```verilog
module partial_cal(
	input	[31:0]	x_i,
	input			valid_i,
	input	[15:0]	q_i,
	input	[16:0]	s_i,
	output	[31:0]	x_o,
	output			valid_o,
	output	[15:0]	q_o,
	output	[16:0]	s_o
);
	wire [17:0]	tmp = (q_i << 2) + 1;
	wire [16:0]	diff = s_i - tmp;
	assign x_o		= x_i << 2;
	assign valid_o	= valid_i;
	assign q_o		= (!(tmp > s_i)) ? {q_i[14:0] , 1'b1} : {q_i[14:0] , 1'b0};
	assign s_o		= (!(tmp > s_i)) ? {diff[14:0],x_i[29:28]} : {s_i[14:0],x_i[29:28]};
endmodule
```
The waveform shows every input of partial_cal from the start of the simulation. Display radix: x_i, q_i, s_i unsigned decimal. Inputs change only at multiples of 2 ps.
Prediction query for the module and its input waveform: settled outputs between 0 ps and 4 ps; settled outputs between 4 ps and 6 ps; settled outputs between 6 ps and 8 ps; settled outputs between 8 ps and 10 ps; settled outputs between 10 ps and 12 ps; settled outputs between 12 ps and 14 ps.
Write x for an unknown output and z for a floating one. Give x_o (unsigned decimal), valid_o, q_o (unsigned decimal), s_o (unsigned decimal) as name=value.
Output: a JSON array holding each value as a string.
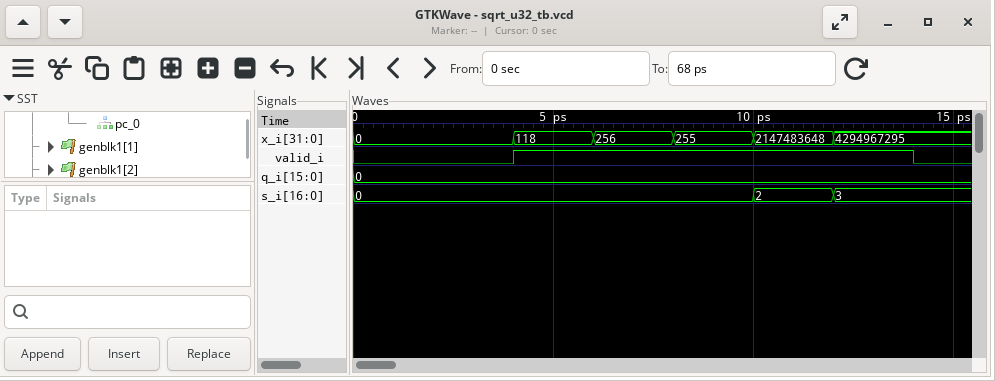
["x_o=0, valid_o=0, q_o=0, s_o=0", "x_o=472, valid_o=1, q_o=0, s_o=0", "x_o=1024, valid_o=1, q_o=0, s_o=0", "x_o=1020, valid_o=1, q_o=0, s_o=0", "x_o=0, valid_o=1, q_o=1, s_o=4", "x_o=4294967292, valid_o=1, q_o=1, s_o=11"]
